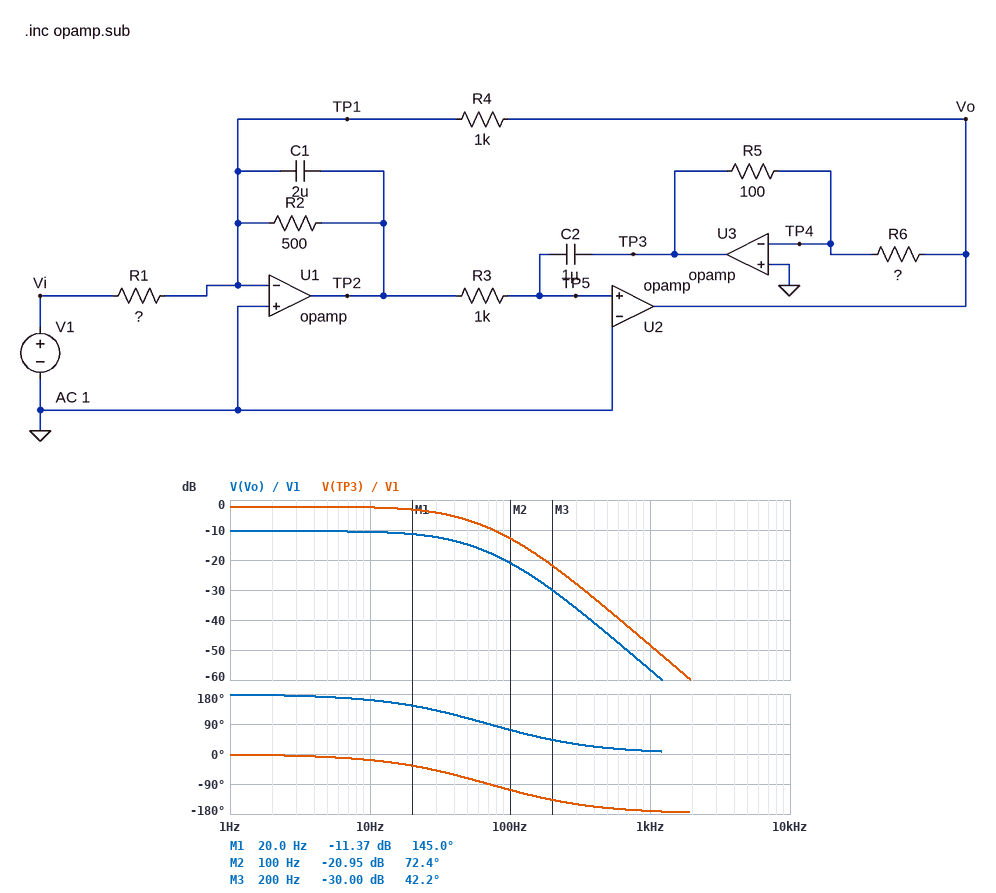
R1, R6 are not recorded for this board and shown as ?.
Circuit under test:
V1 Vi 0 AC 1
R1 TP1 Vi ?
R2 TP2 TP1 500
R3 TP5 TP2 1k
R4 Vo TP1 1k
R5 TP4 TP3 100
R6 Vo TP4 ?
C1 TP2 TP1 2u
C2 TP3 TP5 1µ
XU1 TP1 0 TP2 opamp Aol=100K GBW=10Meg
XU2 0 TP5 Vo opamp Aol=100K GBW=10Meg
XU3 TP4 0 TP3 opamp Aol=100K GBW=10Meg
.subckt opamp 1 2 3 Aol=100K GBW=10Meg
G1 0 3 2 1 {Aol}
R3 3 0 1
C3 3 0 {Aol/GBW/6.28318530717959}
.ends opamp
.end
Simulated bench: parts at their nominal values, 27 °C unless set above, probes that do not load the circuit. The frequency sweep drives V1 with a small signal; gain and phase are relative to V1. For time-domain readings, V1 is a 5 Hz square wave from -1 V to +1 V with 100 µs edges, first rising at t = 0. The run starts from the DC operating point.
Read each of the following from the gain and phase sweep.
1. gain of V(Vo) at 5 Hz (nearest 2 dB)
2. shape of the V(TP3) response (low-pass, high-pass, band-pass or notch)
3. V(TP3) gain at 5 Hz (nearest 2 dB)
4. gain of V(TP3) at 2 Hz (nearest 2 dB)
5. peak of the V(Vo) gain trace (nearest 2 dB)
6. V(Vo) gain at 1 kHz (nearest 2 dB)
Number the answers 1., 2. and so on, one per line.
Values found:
1. -10 dB
2. low-pass
3. -2 dB
4. -2 dB
5. -10 dB
6. -56 dB
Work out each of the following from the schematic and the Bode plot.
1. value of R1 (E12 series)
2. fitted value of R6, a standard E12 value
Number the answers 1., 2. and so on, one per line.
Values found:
1. 3.3 kΩ
2. 39 Ω
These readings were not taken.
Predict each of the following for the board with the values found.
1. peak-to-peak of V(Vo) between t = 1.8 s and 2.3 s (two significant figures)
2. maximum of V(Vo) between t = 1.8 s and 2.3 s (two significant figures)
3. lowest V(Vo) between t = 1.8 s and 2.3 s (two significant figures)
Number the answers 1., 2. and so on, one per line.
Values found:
1. 610 mV
2. 300 mV
3. -300 mV
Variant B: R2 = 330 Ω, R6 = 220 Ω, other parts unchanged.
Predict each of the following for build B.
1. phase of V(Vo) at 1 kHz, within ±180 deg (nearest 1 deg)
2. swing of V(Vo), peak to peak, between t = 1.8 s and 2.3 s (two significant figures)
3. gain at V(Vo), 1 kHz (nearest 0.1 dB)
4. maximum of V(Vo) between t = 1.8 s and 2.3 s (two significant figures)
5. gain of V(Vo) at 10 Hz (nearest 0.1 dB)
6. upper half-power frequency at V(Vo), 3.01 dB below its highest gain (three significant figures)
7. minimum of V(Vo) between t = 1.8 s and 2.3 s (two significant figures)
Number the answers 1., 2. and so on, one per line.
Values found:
1. 14 deg
2. 660 mV
3. -41.5 dB
4. 330 mV
5. -10.4 dB
6. 163 Hz
7. -330 mV
